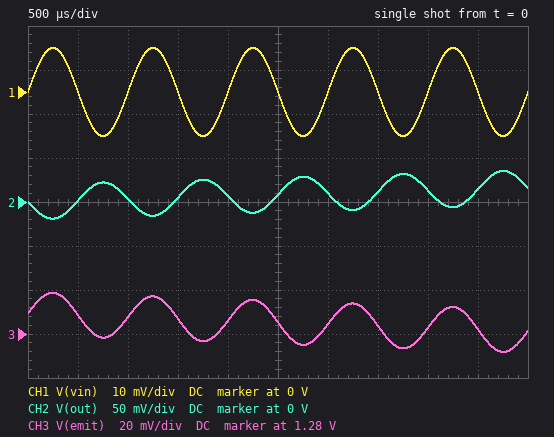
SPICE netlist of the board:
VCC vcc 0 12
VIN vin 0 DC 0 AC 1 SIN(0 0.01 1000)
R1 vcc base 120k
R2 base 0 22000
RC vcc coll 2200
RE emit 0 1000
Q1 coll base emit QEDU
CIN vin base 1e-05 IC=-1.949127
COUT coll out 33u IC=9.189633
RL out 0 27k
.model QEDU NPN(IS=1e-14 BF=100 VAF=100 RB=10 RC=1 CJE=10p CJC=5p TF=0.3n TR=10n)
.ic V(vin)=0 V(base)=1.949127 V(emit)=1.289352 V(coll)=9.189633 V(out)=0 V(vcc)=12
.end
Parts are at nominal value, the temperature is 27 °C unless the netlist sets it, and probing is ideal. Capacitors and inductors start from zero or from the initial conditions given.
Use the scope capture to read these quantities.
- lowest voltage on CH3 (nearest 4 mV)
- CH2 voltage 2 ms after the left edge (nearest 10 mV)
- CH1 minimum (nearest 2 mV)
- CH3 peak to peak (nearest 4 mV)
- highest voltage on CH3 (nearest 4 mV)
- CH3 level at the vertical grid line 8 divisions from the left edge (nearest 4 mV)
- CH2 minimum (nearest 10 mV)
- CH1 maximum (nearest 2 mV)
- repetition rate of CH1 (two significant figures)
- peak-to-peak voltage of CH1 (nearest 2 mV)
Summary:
1.272 V
10 mV
-10 mV
28 mV
1.300 V
1.284 V
-20 mV
10 mV
1.0 kHz
20 mV
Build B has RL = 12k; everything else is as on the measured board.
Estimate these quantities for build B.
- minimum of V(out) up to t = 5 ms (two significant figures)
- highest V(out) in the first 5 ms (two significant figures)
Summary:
-17 mV
32 mV
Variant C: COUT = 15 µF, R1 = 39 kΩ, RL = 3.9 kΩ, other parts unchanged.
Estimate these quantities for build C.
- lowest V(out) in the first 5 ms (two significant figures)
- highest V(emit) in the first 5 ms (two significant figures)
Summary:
-100 mV
1.4 V
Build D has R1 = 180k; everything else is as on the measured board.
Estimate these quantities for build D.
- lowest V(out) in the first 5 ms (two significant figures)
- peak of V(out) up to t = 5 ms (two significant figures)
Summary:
-18 mV
61 mV
